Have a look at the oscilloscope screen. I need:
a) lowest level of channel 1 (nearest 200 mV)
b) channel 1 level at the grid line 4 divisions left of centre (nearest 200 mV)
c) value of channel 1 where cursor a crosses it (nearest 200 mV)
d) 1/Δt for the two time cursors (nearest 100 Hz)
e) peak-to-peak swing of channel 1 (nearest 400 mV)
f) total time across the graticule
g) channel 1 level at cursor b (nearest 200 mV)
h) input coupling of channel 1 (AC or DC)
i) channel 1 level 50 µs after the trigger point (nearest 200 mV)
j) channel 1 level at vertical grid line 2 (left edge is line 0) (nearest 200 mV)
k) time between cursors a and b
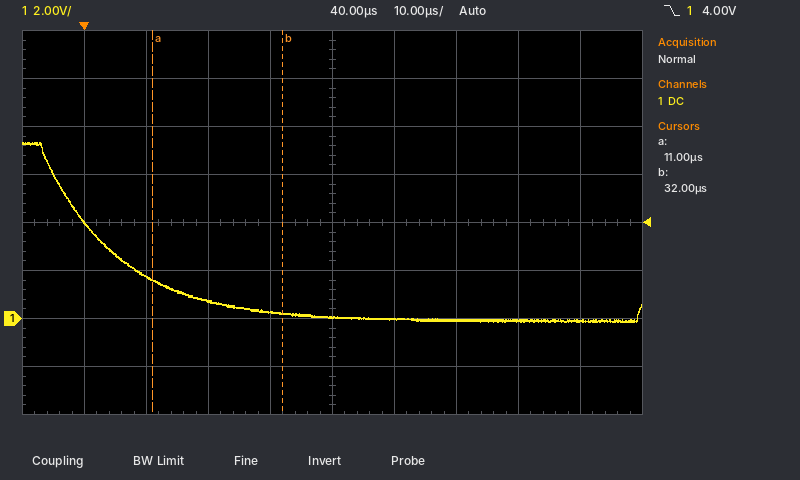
-200 mV
4.0 V
1.6 V
47.6 kHz
7.6 V
100 µs
200 mV
DC
0.0 V
1.8 V
21 µs
